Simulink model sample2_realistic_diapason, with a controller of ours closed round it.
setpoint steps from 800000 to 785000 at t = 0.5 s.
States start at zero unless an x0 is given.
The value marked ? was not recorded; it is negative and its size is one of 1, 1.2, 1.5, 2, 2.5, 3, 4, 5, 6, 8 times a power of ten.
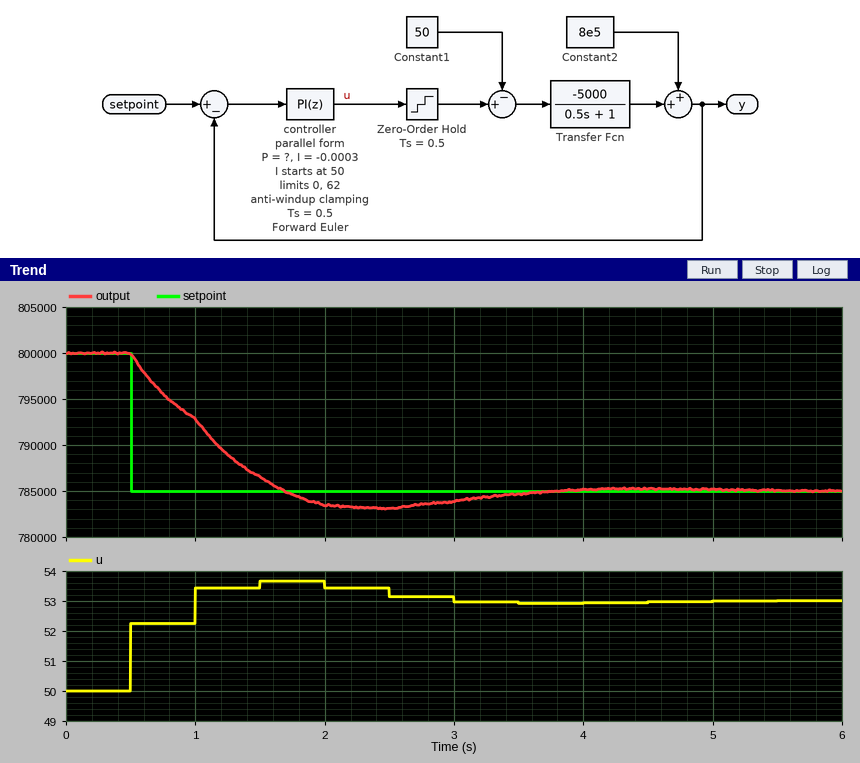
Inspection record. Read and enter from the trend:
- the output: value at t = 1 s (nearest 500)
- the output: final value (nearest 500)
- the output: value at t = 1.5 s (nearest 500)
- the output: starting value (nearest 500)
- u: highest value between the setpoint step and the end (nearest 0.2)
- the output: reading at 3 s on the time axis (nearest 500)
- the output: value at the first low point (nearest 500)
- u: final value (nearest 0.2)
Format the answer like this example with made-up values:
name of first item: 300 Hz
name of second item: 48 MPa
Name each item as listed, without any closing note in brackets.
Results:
the output: value at t = 1 s: 793000
the output: final value: 785000
the output: value at t = 1.5 s: 786500
the output: starting value: 800000
u: highest value between the setpoint step and the end: 53.6
the output: reading at 3 s on the time axis: 784000
the output: value at the first low point: 783000
u: final value: 53.0
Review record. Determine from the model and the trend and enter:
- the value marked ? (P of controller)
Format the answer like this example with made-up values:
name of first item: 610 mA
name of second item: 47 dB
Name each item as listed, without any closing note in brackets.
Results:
the value marked ?: -0.00015
